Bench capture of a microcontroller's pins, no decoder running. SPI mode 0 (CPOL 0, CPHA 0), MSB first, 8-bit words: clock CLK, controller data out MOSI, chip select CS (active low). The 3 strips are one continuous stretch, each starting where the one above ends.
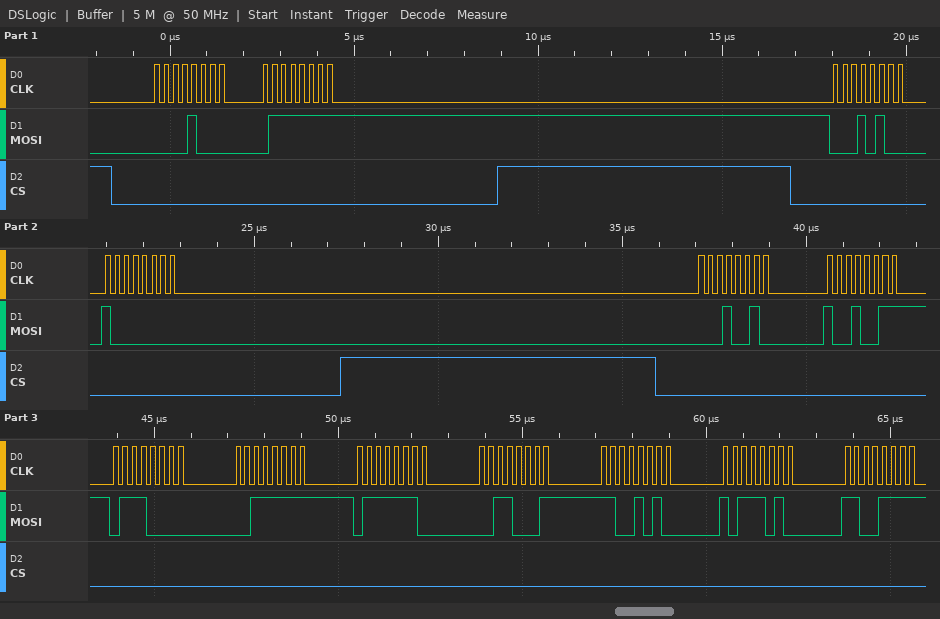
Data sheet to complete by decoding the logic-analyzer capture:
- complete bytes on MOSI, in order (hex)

0x08 0x7F 0x14 0x80 0x12 0x93 0x70 0x3F 0x7E 0x31 0xCA 0xBA 0xCF
